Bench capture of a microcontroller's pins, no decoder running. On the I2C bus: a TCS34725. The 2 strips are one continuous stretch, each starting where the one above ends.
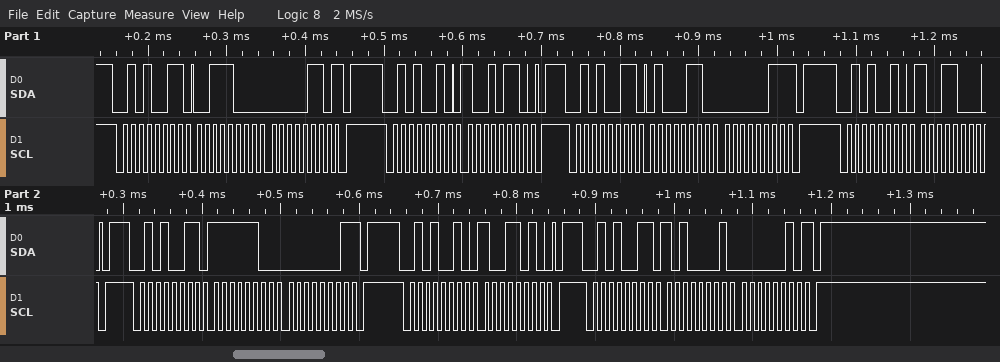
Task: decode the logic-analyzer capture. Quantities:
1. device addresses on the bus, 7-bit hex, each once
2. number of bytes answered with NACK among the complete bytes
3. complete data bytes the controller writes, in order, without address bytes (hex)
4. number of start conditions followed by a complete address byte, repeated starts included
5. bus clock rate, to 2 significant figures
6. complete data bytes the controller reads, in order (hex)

0x29
4
96 98 9A
7
100 kHz
38 06 46 03 FC 01 A1 02
